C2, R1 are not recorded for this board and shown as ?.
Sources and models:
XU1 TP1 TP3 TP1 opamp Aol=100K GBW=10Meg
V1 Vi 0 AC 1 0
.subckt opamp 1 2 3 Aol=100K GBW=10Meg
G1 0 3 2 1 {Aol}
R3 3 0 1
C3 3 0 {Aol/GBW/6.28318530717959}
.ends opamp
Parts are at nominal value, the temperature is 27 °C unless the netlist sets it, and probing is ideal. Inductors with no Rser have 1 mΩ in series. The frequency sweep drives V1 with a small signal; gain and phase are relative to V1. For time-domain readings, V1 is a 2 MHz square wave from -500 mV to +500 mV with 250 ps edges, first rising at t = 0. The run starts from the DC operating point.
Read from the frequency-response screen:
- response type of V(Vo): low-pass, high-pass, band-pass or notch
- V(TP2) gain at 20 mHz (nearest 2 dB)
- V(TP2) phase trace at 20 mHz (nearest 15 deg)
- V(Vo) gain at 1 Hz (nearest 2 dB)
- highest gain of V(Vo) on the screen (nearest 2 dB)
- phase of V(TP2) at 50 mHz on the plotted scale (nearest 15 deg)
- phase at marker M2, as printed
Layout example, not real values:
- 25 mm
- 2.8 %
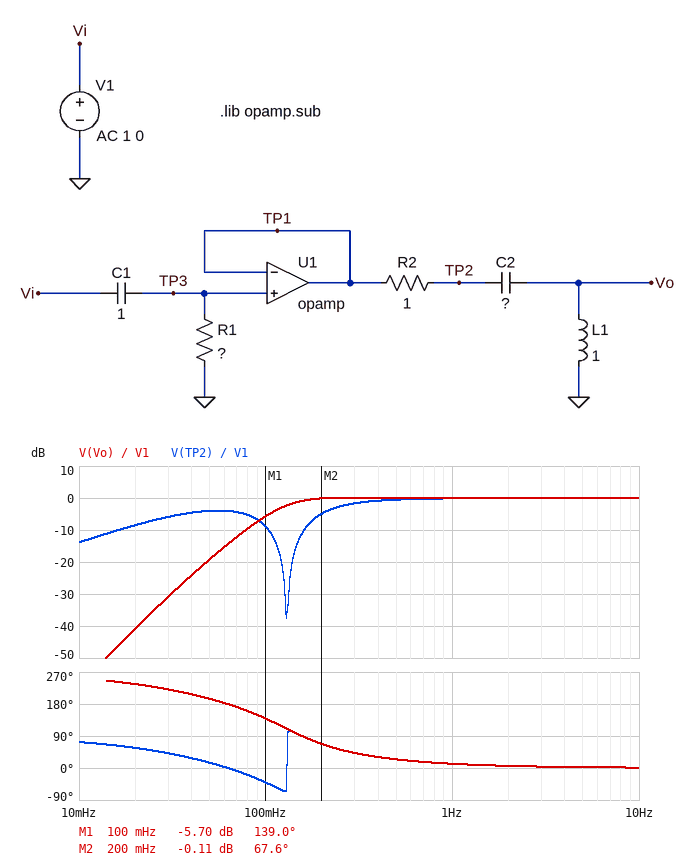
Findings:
- high-pass
- -8 dB
- 60 deg
- 0 dB
- 0 dB
- 15 deg
- 67.6 deg
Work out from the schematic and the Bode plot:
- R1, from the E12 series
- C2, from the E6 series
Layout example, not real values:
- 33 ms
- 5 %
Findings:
- 3.3 Ω
- 1.5 F
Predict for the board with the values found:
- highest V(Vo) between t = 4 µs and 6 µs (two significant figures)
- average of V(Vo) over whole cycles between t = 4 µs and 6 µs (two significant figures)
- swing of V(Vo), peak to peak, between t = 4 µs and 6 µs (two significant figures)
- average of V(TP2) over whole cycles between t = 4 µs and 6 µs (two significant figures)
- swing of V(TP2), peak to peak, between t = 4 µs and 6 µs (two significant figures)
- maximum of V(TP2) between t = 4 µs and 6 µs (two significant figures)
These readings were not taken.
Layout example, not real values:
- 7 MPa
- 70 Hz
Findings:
- 1.0 V
- 500 mV
- 1.0 V
- 500 mV
- 1.0 V
- 1.0 V
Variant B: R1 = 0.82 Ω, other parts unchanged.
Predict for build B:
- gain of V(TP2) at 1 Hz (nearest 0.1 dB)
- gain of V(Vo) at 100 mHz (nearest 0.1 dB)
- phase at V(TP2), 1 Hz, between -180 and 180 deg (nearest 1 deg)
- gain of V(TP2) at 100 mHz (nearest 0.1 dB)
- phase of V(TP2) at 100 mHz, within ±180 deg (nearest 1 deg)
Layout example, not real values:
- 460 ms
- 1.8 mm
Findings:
- -0.3 dB
- -11.6 dB
- 20 deg
- -14.8 dB
- -4 deg
